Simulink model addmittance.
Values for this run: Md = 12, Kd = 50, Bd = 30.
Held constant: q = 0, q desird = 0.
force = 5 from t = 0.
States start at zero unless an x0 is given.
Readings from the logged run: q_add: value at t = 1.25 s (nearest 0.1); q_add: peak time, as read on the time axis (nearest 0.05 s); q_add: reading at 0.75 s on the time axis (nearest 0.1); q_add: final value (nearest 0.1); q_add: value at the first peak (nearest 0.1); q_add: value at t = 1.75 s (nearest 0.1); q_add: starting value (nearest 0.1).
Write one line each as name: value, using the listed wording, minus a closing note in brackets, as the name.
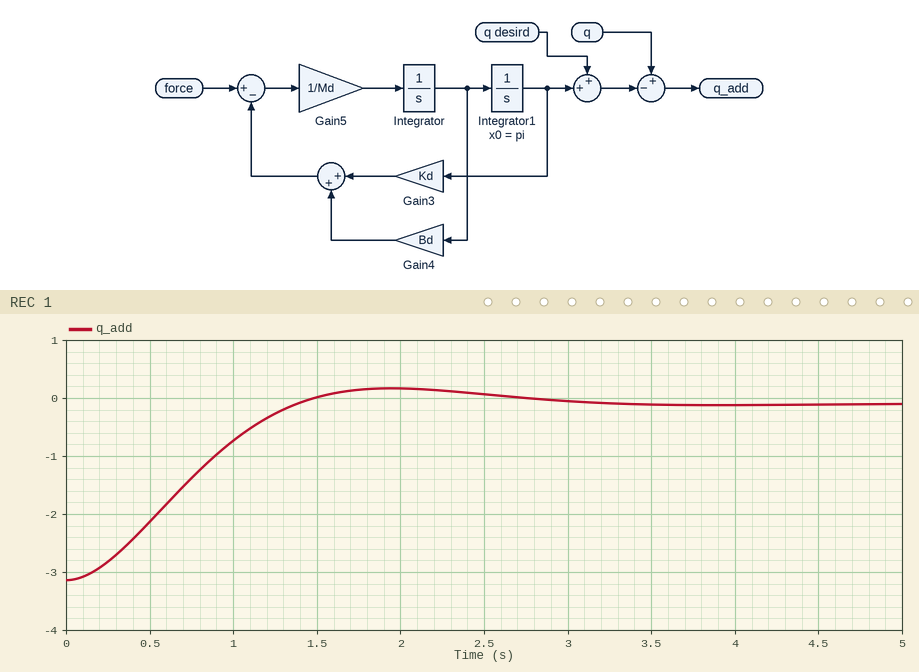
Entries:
q_add: value at t = 1.25 s: -0.3
q_add: peak time, as read on the time axis: 1.95 s
q_add: reading at 0.75 s on the time axis: -1.4
q_add: final value: -0.1
q_add: value at the first peak: 0.2
q_add: value at t = 1.75 s: 0.1
q_add: starting value: -3.1
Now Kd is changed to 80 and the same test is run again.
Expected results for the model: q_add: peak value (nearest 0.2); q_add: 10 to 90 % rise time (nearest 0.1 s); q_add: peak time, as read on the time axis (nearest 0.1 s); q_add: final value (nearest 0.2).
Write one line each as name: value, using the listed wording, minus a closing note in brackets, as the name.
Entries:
q_add: peak value: 0.4
q_add: 10 to 90 % rise time: 0.6 s
q_add: peak time, as read on the time axis: 1.4 s
q_add: final value: 0.0
